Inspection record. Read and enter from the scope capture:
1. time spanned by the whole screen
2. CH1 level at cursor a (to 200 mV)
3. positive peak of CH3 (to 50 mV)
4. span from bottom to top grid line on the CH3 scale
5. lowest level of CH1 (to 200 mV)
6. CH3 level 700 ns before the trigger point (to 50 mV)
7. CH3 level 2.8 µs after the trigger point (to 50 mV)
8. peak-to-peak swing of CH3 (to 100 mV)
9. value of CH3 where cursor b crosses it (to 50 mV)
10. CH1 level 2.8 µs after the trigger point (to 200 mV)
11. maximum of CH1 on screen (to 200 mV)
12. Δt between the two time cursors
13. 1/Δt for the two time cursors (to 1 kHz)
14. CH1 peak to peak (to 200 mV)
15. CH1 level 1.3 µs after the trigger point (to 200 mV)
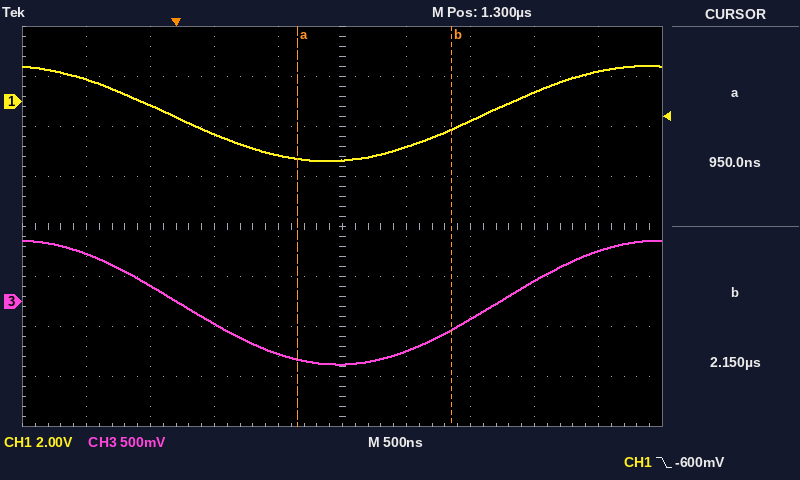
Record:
5 µs
-2.2 V
600 mV
4 V
-2.4 V
500 mV
200 mV
1.20 V
-300 mV
400 mV
1.4 V
1.20 µs
833 kHz
3.8 V
-2.4 V
